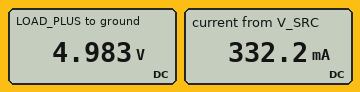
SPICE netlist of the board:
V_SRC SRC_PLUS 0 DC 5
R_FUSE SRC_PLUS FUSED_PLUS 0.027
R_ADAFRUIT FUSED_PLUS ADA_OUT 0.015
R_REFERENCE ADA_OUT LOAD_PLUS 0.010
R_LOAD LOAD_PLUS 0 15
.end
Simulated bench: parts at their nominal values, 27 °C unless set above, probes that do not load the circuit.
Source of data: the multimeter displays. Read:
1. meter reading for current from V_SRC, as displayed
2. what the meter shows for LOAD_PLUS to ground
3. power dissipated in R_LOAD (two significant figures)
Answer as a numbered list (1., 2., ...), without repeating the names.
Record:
1. 332.2 mA
2. 4.983 V
3. 1.7 W
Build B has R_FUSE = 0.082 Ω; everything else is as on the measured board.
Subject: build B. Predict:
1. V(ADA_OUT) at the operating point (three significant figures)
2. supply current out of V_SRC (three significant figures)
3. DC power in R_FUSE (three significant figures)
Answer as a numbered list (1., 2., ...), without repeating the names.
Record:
1. 4.97 V
2. 331 mA
3. 8.98 mW
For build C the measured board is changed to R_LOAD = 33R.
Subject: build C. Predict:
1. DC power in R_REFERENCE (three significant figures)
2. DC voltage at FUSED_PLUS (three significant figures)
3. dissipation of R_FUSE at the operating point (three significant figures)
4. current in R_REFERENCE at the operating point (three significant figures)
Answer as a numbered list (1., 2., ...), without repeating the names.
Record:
1. 229 µW
2. 5.00 V
3. 618 µW
4. 151 mA
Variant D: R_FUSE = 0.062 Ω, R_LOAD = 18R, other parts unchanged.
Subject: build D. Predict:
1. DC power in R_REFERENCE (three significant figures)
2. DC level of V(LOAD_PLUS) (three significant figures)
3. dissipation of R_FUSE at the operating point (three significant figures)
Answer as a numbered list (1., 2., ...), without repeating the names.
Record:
1. 764 µW
2. 4.98 V
3. 4.74 mW
